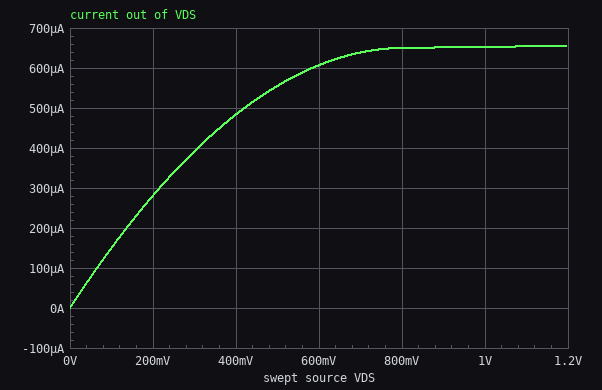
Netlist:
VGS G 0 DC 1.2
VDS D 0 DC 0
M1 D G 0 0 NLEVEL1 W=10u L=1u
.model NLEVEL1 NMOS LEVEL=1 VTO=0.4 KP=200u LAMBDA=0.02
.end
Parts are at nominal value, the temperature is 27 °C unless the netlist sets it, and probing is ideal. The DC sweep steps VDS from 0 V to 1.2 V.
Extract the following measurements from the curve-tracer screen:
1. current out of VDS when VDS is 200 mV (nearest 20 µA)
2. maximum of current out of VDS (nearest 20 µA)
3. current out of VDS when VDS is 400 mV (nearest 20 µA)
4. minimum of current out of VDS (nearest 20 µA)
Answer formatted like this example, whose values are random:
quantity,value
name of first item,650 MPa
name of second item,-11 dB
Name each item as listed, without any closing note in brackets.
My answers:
quantity,value
current out of VDS when VDS is 200 mV,280 µA
maximum of current out of VDS,660 µA
current out of VDS when VDS is 400 mV,480 µA
minimum of current out of VDS,0 A
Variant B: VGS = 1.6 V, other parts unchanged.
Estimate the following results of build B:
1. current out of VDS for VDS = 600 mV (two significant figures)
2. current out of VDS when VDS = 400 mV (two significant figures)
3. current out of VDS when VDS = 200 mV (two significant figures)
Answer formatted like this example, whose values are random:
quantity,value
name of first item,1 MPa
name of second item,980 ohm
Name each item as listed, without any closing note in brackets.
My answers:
quantity,value
current out of VDS for VDS = 600 mV,1.1 mA
current out of VDS when VDS = 400 mV,810 µA
current out of VDS when VDS = 200 mV,440 µA
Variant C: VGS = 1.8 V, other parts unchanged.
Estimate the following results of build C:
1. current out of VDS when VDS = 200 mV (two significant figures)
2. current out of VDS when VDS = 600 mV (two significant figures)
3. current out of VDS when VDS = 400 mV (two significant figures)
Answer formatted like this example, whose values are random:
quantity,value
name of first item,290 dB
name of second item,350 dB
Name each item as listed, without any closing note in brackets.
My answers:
quantity,value
current out of VDS when VDS = 200 mV,520 µA
current out of VDS when VDS = 600 mV,1.3 mA
current out of VDS when VDS = 400 mV,970 µA
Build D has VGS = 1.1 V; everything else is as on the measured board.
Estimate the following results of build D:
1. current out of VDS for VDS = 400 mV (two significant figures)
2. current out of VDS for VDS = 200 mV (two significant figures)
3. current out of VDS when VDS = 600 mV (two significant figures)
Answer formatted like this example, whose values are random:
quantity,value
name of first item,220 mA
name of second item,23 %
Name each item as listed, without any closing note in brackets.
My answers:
quantity,value
current out of VDS for VDS = 400 mV,400 µA
current out of VDS for VDS = 200 mV,240 µA
current out of VDS when VDS = 600 mV,490 µA
